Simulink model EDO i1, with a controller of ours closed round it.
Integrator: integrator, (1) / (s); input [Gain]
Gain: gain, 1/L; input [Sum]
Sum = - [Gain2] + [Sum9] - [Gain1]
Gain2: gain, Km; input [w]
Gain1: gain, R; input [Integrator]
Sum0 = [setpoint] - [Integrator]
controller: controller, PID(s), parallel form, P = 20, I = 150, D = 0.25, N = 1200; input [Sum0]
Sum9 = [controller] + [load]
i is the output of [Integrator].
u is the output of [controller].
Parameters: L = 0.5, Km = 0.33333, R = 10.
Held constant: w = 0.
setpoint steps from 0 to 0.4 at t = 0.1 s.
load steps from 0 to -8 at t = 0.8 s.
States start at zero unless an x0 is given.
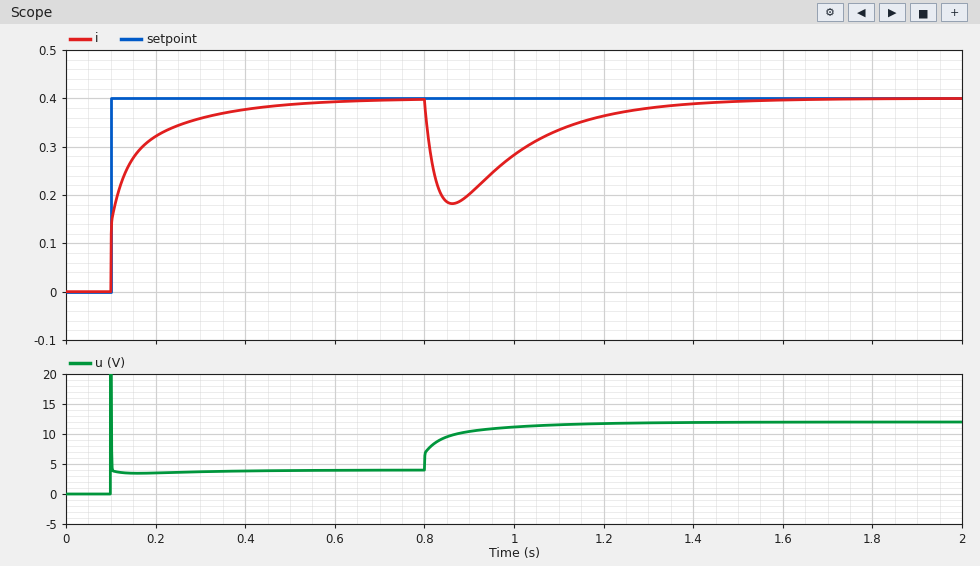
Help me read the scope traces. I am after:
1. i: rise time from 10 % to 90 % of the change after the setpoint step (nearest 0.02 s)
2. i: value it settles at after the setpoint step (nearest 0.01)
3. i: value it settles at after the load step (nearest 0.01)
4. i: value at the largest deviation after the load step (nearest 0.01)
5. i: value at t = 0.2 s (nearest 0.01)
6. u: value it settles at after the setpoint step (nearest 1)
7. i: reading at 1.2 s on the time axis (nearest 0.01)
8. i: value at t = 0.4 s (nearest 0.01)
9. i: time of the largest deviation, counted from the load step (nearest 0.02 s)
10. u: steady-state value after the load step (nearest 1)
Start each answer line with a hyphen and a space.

- 0.20 s
- 0.40
- 0.40
- 0.18
- 0.32
- 4
- 0.36
- 0.38
- 0.06 s
- 12
